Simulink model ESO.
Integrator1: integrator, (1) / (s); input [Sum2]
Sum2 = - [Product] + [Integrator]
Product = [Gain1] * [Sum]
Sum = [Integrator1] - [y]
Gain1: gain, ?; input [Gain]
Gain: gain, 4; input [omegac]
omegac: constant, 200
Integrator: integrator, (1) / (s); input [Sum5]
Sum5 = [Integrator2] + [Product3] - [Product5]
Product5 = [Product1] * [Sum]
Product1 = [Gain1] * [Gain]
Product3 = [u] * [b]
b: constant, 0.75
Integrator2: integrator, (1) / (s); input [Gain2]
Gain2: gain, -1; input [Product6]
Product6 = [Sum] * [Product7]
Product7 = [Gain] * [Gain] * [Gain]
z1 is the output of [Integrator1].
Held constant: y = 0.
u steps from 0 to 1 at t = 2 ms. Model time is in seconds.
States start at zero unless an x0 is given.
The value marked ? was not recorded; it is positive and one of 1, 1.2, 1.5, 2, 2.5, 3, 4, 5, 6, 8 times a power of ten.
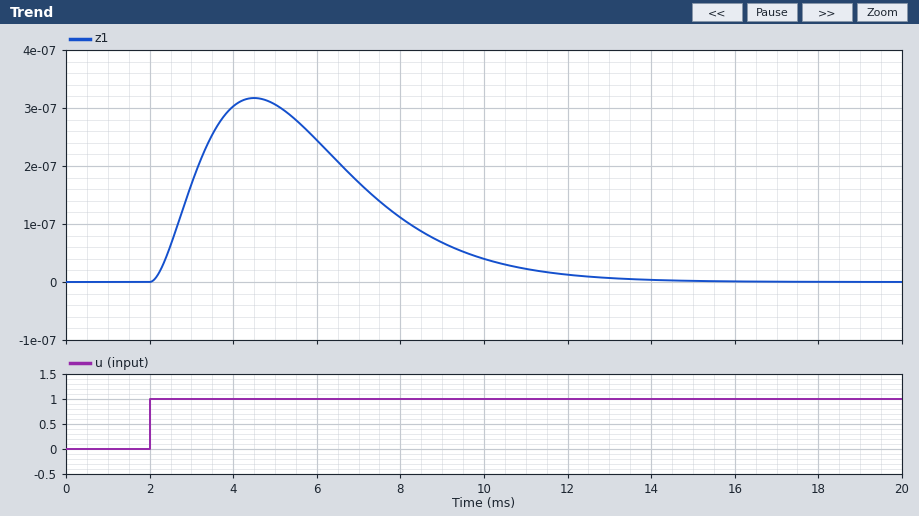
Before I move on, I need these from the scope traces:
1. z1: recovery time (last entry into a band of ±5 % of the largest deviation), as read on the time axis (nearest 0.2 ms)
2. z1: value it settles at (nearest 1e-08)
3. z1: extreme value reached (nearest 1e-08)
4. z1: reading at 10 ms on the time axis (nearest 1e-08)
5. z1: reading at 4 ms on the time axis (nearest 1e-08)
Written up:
11.6 ms
0.00000000
0.00000032
0.00000004
0.00000030
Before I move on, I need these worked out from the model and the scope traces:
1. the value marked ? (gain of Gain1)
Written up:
3
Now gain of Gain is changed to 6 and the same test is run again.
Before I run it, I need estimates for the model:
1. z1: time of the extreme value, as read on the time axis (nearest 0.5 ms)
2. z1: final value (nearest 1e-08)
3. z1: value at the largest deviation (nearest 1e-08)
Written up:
3.5 ms
0.00000000
0.00000014
